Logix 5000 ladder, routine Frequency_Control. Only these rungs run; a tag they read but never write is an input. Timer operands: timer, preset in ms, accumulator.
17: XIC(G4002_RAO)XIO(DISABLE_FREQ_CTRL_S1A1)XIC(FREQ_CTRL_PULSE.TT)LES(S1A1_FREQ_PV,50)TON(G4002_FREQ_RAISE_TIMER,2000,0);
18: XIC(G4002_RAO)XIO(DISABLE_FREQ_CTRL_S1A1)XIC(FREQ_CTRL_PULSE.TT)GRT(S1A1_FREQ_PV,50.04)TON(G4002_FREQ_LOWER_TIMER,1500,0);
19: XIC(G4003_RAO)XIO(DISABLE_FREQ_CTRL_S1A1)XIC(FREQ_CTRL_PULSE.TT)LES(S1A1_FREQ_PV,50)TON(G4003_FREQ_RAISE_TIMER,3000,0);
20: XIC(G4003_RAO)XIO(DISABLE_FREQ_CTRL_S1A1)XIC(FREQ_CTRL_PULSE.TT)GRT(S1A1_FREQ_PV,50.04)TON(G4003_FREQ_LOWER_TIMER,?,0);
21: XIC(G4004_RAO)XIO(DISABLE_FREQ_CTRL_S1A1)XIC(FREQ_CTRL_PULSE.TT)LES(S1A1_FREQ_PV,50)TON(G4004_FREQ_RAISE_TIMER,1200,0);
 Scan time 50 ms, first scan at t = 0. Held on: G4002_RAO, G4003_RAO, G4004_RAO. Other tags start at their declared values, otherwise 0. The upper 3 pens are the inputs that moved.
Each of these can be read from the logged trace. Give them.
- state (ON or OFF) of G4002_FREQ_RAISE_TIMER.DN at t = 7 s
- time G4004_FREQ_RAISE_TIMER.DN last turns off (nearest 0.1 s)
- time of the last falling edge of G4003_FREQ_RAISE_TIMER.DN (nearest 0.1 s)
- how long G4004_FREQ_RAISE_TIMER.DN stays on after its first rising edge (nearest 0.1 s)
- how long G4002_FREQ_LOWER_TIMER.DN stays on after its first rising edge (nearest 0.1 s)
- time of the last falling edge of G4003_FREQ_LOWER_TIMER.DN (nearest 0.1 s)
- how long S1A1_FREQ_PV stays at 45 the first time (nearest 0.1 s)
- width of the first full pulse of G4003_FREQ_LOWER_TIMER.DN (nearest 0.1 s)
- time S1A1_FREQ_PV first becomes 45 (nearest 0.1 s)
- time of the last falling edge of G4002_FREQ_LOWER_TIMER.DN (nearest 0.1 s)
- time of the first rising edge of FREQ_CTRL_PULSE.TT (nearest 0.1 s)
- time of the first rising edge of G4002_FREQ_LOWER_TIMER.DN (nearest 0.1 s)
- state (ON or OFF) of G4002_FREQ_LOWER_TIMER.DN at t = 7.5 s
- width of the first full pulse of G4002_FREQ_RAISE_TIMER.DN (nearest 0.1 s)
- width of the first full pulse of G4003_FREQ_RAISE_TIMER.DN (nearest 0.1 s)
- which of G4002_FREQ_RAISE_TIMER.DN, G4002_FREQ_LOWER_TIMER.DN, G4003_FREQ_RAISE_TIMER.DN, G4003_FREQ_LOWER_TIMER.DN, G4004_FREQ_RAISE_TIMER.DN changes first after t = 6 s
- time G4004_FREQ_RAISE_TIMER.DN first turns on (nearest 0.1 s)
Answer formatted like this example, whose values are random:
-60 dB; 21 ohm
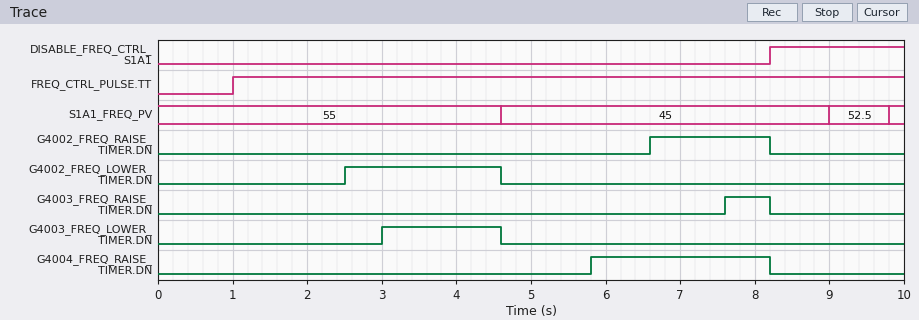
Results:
ON; 8.2 s; 8.2 s; 2.4 s; 2.1 s; 4.6 s; 4.4 s; 1.6 s; 4.6 s; 4.6 s; 1.0 s; 2.5 s; OFF; 1.6 s; 0.6 s; G4002_FREQ_RAISE_TIMER.DN; 5.8 s
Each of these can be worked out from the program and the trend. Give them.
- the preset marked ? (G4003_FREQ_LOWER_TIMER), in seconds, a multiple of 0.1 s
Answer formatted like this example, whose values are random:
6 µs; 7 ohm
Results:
2.0 s
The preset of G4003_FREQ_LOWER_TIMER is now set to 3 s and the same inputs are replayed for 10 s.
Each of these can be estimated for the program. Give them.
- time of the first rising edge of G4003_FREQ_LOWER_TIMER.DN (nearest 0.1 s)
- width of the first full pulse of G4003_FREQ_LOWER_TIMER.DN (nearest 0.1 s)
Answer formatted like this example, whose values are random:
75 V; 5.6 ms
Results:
4.0 s; 0.6 s
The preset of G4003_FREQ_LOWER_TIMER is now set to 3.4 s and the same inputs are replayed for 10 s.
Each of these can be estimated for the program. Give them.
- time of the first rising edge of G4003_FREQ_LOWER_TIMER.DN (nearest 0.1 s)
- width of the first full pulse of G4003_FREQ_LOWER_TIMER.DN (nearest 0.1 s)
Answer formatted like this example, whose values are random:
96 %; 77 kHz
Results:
4.4 s; 0.2 s
